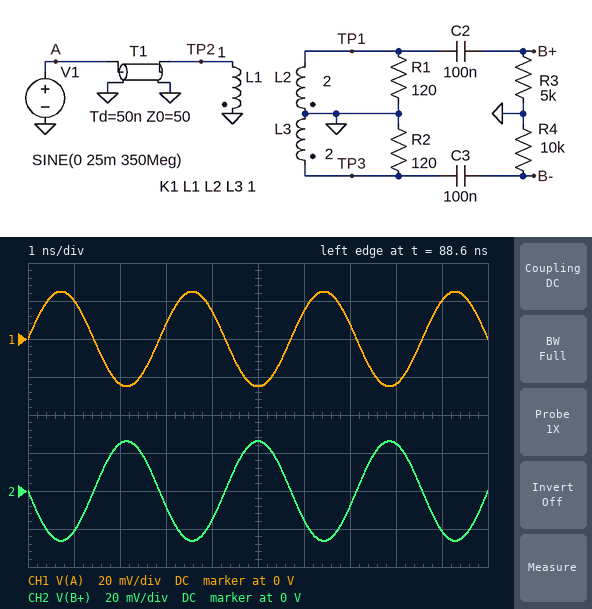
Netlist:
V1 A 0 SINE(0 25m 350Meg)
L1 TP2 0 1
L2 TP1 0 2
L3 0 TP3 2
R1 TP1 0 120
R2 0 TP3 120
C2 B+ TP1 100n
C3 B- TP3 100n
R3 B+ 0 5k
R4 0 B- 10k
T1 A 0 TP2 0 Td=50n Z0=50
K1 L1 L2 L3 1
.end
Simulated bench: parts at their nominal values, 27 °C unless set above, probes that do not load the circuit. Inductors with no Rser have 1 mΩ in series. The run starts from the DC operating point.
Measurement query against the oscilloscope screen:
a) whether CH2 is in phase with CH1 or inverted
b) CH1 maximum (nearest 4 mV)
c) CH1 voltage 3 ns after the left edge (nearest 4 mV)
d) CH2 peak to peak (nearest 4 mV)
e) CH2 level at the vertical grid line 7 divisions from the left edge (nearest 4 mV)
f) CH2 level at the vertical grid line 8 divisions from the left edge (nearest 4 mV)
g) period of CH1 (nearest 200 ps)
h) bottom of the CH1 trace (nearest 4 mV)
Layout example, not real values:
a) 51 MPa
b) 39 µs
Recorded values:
a) inverted
b) 24 mV
c) 8 mV
d) 52 mV
e) -8 mV
f) 24 mV
g) 2.8 ns
h) -24 mV
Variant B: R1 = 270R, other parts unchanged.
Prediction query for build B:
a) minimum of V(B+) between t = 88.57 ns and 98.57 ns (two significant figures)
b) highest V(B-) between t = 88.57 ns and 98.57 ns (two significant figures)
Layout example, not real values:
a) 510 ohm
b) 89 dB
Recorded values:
a) -32 mV
b) 32 mV
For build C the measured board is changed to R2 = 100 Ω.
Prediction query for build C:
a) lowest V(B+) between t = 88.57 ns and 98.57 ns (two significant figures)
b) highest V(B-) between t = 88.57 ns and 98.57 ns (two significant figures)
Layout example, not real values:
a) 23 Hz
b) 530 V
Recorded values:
a) -25 mV
b) 25 mV
